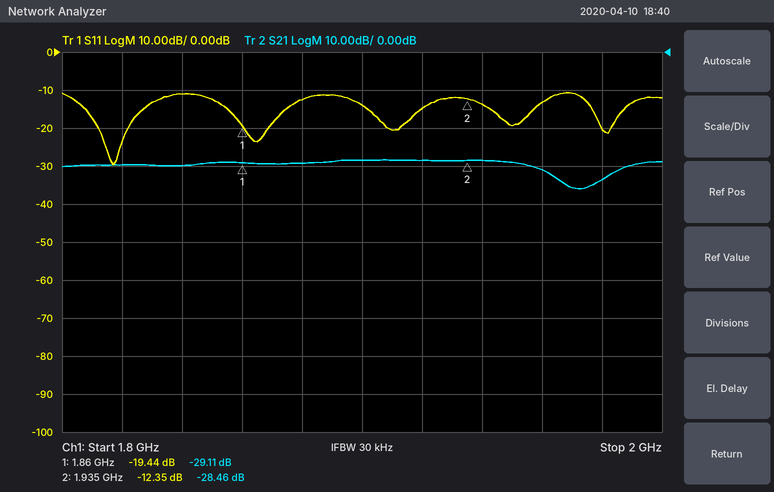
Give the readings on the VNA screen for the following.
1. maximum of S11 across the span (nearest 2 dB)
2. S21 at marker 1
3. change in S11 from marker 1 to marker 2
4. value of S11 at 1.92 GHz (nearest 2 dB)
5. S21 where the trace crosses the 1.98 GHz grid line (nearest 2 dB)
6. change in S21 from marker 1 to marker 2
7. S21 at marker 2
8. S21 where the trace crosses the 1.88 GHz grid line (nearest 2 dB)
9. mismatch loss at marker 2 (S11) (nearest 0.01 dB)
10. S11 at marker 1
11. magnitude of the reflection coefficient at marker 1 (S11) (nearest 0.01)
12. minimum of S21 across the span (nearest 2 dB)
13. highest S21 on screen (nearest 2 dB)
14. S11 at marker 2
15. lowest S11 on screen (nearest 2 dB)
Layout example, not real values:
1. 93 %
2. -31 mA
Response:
1. -10 dB
2. -29.11 dB
3. 7.09 dB
4. -14 dB
5. -34 dB
6. 0.65 dB
7. -28.46 dB
8. -30 dB
9. 0.26 dB
10. -19.44 dB
11. 0.11
12. -36 dB
13. -28 dB
14. -12.35 dB
15. -30 dB
